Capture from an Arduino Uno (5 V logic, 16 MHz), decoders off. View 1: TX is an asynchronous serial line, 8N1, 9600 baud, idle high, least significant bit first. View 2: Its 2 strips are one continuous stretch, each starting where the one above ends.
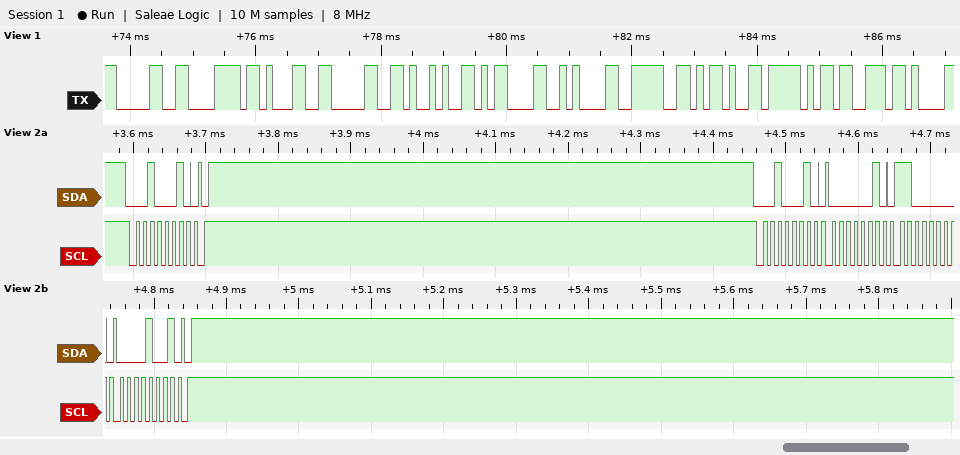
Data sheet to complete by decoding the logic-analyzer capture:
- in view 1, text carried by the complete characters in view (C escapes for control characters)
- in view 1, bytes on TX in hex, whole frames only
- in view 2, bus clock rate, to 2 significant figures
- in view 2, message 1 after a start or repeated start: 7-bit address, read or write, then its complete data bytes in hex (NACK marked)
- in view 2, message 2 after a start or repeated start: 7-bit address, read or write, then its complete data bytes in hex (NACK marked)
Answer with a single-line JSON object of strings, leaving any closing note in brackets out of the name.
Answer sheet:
{"in view 1, text carried by the complete characters in view": "\"0x10)\\r\\n>-_s\"", "in view 1, bytes on TX in hex, whole frames only": "0x30 0x78 0x31 0x30 0x29 0x0D 0x0A 0x3E 0x2D 0x5F 0x73", "in view 2, bus clock rate, to 2 significant figures": "100 kHz", "in view 2, message 1 after a start or repeated start: 7-bit address, read or write, then its complete data bytes in hex": "0x11 write", "in view 2, message 2 after a start or repeated start: 7-bit address, read or write, then its complete data bytes in hex": "0x11 write: 02 C0 09"}
